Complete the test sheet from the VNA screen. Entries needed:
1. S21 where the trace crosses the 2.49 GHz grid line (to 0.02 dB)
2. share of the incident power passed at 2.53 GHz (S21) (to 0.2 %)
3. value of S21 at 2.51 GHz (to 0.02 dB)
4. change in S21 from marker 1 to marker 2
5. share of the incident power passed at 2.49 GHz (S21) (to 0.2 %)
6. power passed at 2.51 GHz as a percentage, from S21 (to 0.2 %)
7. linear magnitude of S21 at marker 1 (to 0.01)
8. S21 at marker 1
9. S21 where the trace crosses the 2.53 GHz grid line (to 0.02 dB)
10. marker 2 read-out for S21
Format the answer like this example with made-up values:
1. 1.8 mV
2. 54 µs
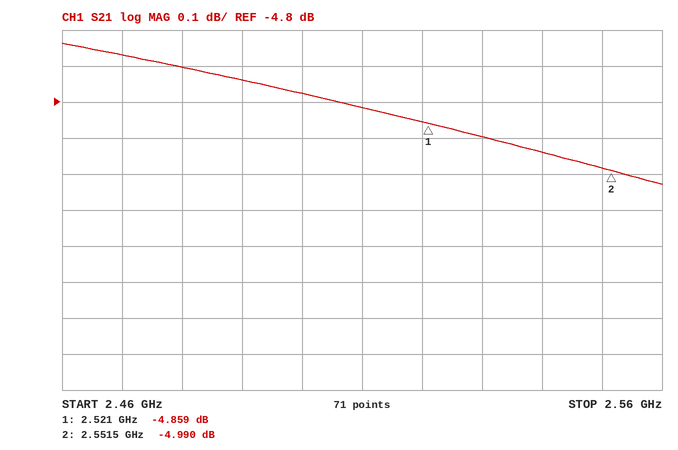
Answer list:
1. -4.74 dB
2. 32.4 %
3. -4.82 dB
4. -0.131 dB
5. 33.6 %
6. 33.0 %
7. 0.57
8. -4.859 dB
9. -4.90 dB
10. -4.990 dB
